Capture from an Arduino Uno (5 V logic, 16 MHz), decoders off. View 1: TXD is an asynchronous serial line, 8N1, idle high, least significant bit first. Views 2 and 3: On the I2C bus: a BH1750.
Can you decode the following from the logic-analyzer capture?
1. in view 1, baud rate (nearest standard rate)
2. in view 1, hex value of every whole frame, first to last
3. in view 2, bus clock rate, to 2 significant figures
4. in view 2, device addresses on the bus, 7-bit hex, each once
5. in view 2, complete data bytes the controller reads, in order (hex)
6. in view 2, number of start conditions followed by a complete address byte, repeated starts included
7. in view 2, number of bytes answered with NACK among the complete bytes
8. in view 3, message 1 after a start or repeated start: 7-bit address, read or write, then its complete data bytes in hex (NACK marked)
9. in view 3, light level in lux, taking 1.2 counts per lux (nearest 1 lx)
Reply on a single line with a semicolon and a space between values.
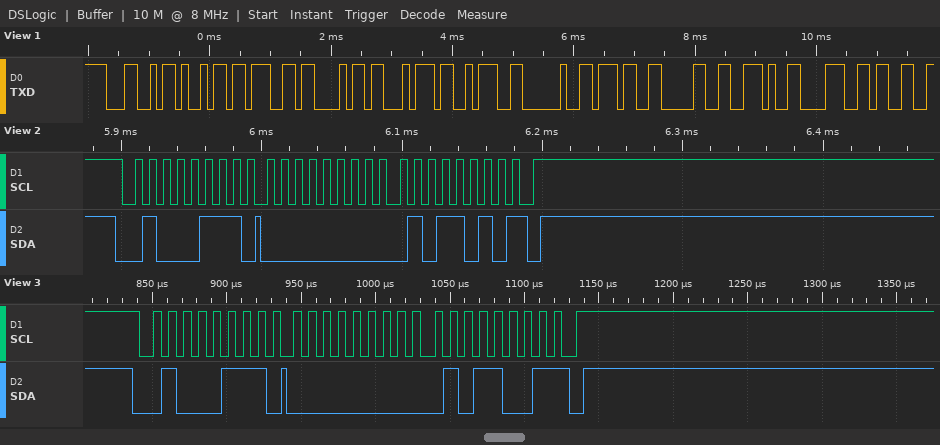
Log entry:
9600 baud; 0x4C 0x69 0x67 0x68 0x74 0x3A 0x20 0x37 0x30 0x2E 0x38 0x33; 100 kHz; 0x23; 00 5A; 1; 1; 0x23 read: 00 59 NACK; 74 lx
